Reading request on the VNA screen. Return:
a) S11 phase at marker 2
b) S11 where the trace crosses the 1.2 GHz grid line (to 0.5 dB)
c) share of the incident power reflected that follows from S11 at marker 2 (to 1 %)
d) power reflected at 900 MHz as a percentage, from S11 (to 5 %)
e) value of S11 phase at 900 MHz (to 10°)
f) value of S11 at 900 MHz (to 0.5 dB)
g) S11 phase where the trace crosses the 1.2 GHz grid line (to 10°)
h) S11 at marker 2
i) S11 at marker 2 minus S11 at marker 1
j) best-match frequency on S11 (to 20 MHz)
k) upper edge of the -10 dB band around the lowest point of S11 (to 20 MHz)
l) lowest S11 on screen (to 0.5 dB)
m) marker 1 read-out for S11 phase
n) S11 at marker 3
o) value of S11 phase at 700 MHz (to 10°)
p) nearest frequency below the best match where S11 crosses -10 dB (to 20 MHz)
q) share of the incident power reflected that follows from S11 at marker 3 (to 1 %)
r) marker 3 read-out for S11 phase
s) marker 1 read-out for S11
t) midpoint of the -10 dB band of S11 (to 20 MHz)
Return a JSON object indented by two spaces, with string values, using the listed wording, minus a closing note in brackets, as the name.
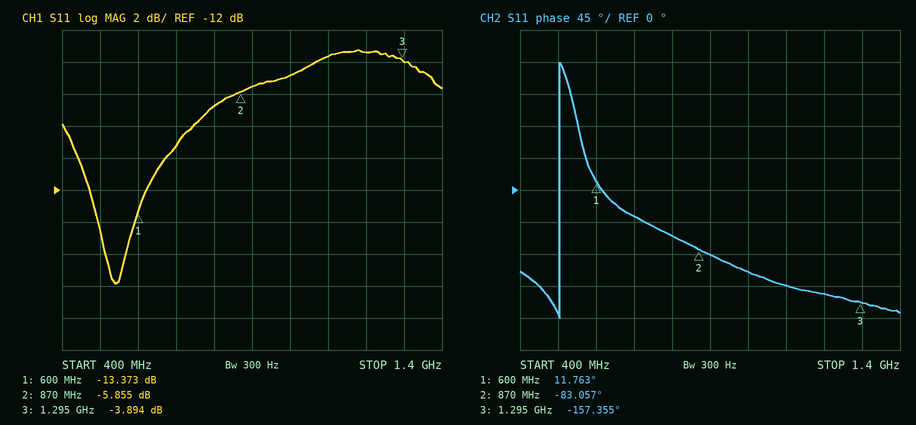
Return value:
{
  "S11 phase at marker 2": "-83.057°",
  "S11 where the trace crosses the 1.2 GHz grid line": "-3.5 dB",
  "share of the incident power reflected that follows from S11 at marker 2": "26 %",
  "power reflected at 900 MHz as a percentage, from S11": "30 %",
  "value of S11 phase at 900 MHz": "-90°",
  "value of S11 at 900 MHz": "-5.5 dB",
  "S11 phase where the trace crosses the 1.2 GHz grid line": "-150°",
  "S11 at marker 2": "-5.855 dB",
  "S11 at marker 2 minus S11 at marker 1": "7.518 dB",
  "best-match frequency on S11": "540 MHz",
  "upper edge of the -10 dB band around the lowest point of S11": "680 MHz",
  "lowest S11 on screen": "-18.0 dB",
  "marker 1 read-out for S11 phase": "11.763°",
  "S11 at marker 3": "-3.894 dB",
  "value of S11 phase at 700 MHz": "-40°",
  "nearest frequency below the best match where S11 crosses -10 dB": "440 MHz",
  "share of the incident power reflected that follows from S11 at marker 3": "41 %",
  "marker 3 read-out for S11 phase": "-157.355°",
  "marker 1 read-out for S11": "-13.373 dB",
  "midpoint of the -10 dB band of S11": "560 MHz"
}
